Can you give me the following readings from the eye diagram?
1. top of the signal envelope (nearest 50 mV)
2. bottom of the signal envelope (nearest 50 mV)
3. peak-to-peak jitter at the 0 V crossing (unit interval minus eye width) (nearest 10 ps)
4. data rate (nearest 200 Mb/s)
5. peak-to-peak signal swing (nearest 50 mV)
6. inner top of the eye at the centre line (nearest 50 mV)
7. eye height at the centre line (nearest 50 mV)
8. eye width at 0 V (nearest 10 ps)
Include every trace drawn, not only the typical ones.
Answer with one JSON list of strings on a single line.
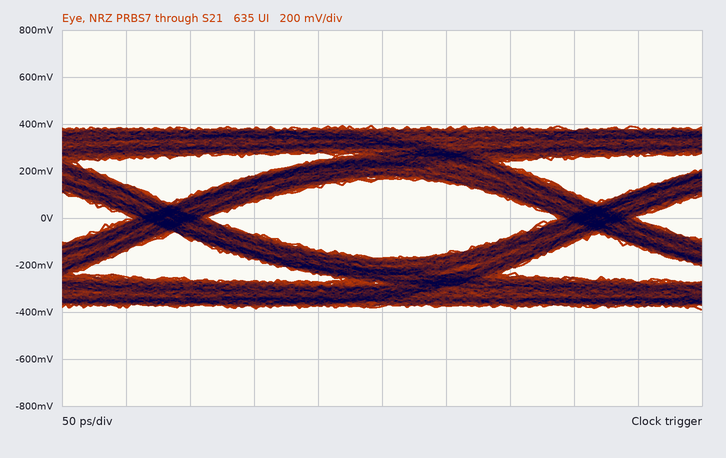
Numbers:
["400 mV", "-400 mV", "60 ps", "3.0 Gb/s", "800 mV", "150 mV", "350 mV", "270 ps"]
